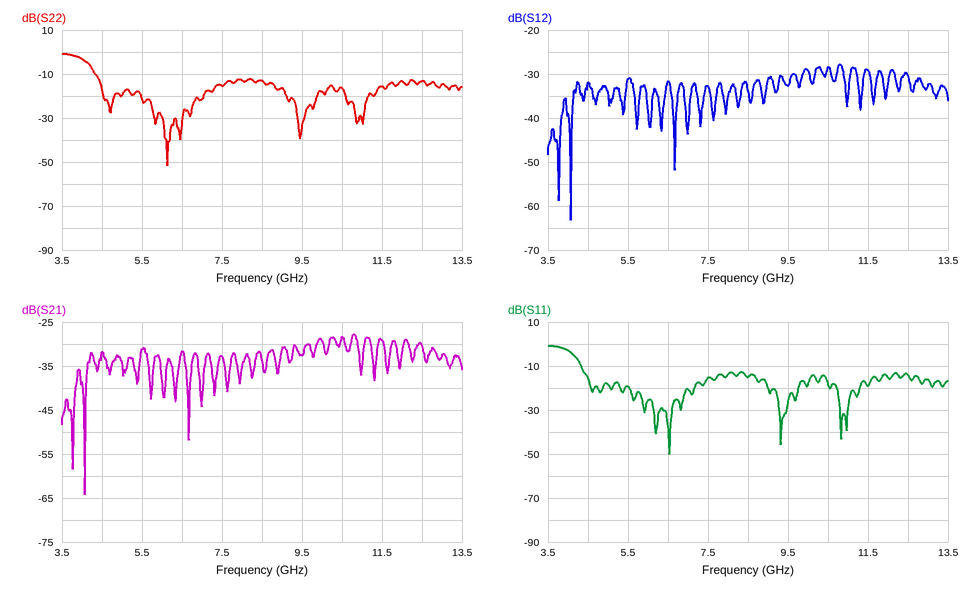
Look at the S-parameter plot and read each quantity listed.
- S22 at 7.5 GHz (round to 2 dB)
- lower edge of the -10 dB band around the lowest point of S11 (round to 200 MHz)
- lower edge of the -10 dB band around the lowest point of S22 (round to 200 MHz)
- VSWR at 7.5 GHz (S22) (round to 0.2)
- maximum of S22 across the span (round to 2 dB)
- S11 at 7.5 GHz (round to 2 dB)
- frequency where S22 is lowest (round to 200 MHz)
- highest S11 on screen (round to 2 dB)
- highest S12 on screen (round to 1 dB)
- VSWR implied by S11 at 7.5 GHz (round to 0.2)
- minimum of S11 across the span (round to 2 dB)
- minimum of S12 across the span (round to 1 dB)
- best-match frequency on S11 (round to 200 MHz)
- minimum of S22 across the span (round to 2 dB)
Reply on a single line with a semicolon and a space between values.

-16 dB; 4.4 GHz; 4.4 GHz; 1.4; 0 dB; -16 dB; 6.2 GHz; 0 dB; -28 dB; 1.4; -50 dB; -63 dB; 6.6 GHz; -52 dB
